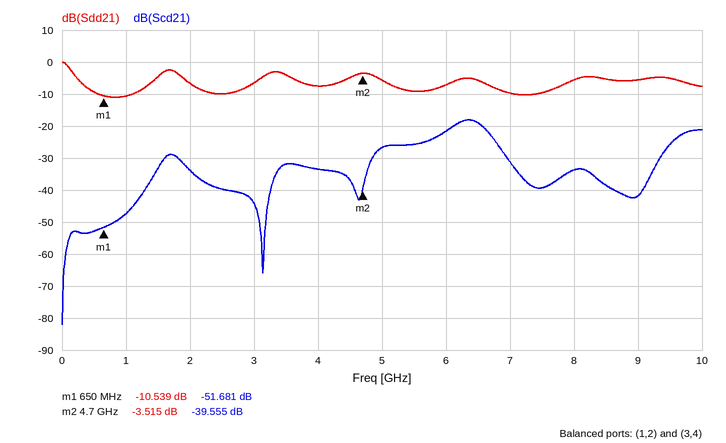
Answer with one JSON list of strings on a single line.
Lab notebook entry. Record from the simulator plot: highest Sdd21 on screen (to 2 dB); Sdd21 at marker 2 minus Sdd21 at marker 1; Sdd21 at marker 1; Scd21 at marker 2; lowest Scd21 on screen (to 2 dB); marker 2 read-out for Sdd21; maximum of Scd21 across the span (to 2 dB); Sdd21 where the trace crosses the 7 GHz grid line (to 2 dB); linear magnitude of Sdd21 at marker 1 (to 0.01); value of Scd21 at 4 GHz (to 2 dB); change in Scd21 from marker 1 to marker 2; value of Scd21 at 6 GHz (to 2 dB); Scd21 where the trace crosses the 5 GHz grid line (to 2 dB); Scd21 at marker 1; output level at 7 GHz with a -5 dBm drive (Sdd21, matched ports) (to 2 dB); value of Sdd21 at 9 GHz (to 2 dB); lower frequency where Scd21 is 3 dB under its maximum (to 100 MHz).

["0 dB", "7.024 dB", "-10.539 dB", "-39.555 dB", "-82 dB", "-3.515 dB", "-18 dB", "-10 dB", "0.30", "-34 dB", "12.126 dB", "-22 dB", "-26 dB", "-51.681 dB", "-14 dBm", "-6 dB", "6.0 GHz"]
